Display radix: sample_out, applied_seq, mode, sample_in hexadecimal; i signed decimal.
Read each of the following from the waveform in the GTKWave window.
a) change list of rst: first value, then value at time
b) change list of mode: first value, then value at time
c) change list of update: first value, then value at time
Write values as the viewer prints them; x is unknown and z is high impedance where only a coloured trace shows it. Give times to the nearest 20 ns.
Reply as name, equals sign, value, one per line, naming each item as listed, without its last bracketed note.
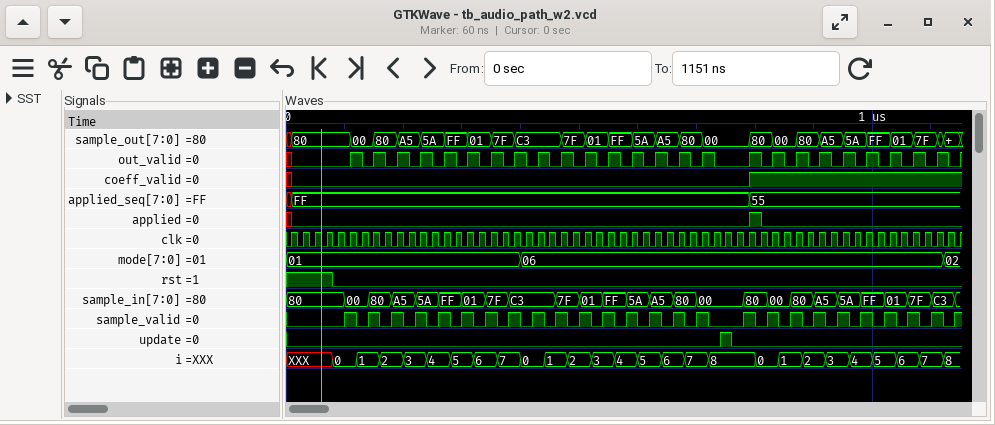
change list of rst: first value, then value at time = 1, 0 at 80 ns
change list of mode: first value, then value at time = 01, 06 at 400 ns, 02 at 1120 ns
change list of update: first value, then value at time = 0, 1 at 740 ns, 0 at 760 ns
